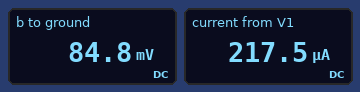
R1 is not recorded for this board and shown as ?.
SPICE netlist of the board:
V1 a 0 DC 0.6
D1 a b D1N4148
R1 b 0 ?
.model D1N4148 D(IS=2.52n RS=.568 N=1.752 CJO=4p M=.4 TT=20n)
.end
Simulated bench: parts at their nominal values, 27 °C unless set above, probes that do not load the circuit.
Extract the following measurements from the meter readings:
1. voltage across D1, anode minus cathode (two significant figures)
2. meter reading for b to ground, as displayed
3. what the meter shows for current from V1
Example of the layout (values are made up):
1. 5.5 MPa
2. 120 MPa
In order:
1. 520 mV
2. 84.8 mV
3. 217.5 µA
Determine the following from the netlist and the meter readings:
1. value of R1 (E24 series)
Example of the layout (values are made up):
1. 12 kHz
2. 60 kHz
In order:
1. 390 Ω
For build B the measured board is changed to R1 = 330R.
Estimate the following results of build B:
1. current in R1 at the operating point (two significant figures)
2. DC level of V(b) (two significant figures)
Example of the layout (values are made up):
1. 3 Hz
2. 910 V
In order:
1. 240 µA
2. 80 mV
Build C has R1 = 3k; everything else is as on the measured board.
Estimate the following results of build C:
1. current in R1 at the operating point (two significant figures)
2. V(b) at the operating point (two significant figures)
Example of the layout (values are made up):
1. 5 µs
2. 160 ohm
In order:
1. 50 µA
2. 150 mV
